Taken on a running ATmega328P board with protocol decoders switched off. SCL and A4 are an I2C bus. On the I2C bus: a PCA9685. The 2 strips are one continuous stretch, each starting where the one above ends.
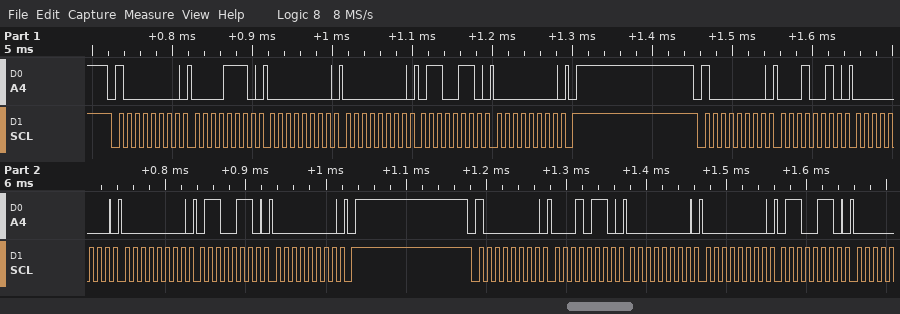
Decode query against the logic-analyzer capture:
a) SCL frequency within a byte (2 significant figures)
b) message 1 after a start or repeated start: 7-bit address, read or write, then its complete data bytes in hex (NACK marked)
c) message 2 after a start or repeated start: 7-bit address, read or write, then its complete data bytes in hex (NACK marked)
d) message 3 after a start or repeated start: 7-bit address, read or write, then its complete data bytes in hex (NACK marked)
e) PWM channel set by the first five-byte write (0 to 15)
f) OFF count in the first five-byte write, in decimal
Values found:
100 kHz
0x40 write: 0E 00 00 66 00
0x40 write: 12 00 00 66 00
0x40 write: 16 00 00 66
2
102
